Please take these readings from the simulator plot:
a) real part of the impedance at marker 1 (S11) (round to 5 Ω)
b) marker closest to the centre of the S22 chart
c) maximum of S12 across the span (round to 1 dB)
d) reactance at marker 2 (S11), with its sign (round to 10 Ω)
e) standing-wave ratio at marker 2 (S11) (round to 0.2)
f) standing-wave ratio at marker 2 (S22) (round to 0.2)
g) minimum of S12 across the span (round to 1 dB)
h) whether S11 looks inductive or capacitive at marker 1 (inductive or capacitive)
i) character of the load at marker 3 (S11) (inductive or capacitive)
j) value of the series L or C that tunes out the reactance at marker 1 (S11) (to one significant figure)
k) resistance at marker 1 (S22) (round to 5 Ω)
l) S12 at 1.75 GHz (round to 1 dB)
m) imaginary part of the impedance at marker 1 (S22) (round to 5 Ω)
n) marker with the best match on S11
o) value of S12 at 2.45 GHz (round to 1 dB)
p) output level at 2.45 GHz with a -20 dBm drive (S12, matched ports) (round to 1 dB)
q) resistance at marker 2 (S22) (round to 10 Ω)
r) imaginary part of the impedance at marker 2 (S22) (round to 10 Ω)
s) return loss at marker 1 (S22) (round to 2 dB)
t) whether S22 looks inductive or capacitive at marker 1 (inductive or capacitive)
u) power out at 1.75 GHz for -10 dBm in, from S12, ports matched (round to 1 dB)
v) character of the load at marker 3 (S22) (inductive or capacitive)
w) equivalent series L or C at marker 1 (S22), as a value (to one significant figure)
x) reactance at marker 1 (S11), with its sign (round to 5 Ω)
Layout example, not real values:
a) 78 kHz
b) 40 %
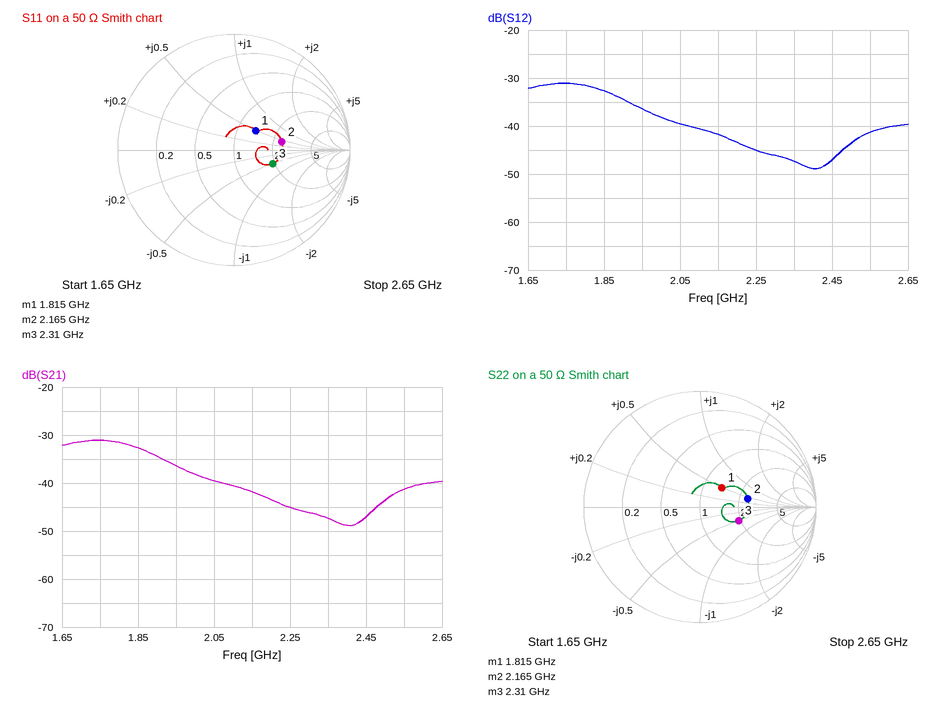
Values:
a) 70 Ω
b) marker 1
c) -31 dB
d) +20 Ω
e) 2.4
f) 2.4
g) -49 dB
h) inductive
i) capacitive
j) 4 pF
k) 70 Ω
l) -31 dB
m) +25 Ω
n) marker 1
o) -47 dB
p) -67 dBm
q) 120 Ω
r) +20 Ω
s) 12 dB
t) inductive
u) -41 dBm
v) capacitive
w) 2 nH
x) +25 Ω
